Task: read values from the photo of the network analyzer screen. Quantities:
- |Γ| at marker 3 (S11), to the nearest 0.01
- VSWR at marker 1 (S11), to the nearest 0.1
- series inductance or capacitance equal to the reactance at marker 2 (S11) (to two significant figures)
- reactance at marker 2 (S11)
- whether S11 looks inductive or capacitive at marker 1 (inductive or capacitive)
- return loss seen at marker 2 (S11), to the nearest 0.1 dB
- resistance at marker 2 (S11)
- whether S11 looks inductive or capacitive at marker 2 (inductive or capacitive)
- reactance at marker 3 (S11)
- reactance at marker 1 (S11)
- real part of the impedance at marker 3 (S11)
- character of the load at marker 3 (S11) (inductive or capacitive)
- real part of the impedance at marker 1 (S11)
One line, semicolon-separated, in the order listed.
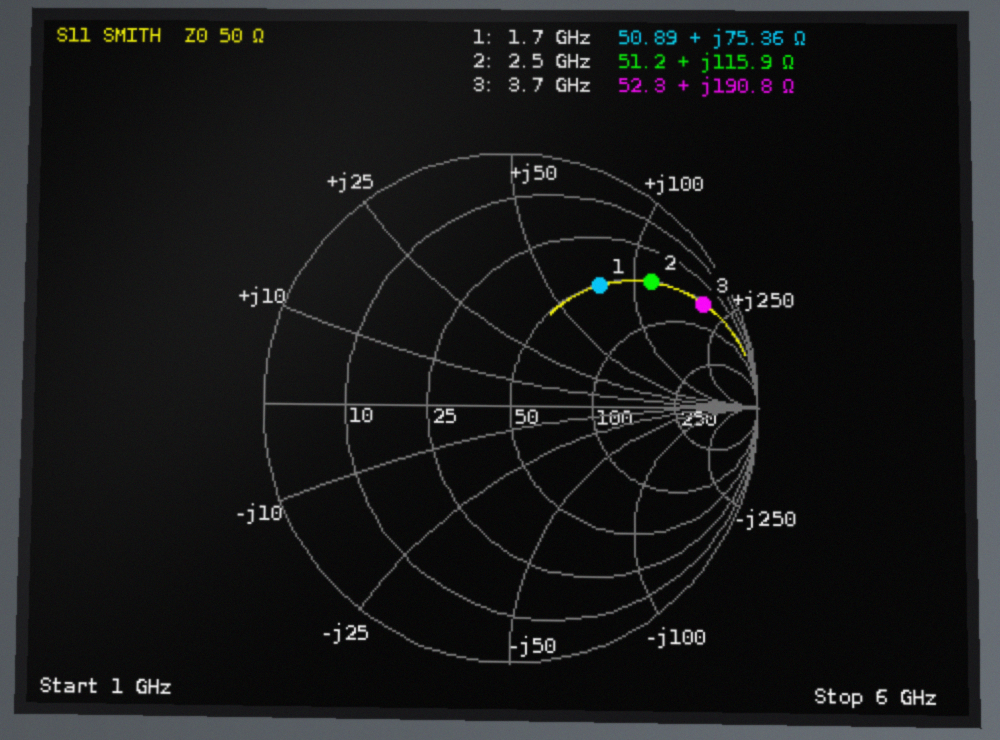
0.88; 4.0; 7.4 nH; +115.9 Ω; inductive; 2.5 dB; 51.2 Ω; inductive; +190.8 Ω; +75.36 Ω; 52.3 Ω; inductive; 50.89 Ω
